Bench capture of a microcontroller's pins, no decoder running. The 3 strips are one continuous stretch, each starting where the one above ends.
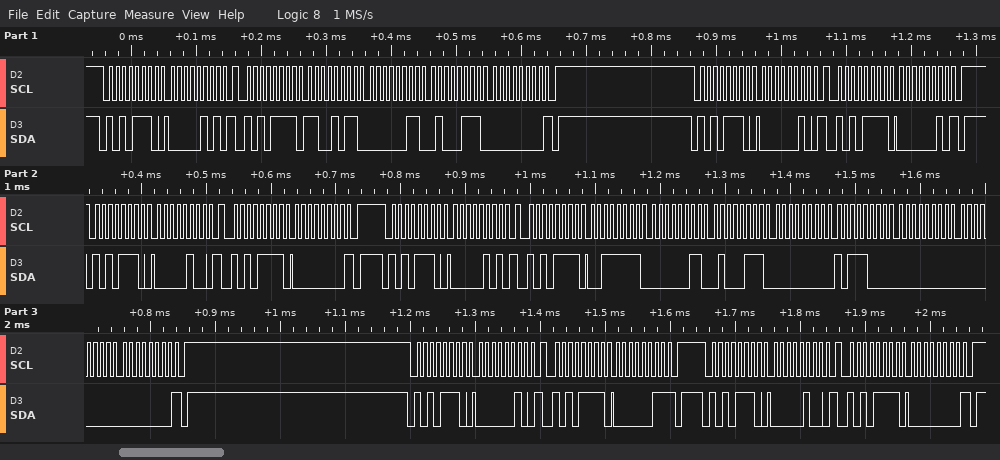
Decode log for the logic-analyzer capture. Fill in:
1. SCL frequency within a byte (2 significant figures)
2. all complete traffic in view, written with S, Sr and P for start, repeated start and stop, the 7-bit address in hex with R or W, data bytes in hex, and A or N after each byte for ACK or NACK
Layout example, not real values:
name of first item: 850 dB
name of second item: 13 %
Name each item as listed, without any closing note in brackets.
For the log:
SCL frequency within a byte: 100 kHz
all complete traffic in view, written with S, Sr and P for start, repeated start and stop, the 7-bit address in hex with R or W, data bytes in hex, and A or N after each byte for ACK or NACK: S 57W A 05 A Sr 57R A CB A 03 A 47 A 00 N P S 57W A 02 A Sr 57R A 02 N P S 57W A 04 A Sr 57R A 00 N P S 57W A 05 A Sr 57R A 3F A 03 A 47 A 00 A B8 A 00 A 00 A 00 N P S 57W A 02 A Sr 57R A 03 N P S 57W A 04 A Sr 57R A 00 N P
